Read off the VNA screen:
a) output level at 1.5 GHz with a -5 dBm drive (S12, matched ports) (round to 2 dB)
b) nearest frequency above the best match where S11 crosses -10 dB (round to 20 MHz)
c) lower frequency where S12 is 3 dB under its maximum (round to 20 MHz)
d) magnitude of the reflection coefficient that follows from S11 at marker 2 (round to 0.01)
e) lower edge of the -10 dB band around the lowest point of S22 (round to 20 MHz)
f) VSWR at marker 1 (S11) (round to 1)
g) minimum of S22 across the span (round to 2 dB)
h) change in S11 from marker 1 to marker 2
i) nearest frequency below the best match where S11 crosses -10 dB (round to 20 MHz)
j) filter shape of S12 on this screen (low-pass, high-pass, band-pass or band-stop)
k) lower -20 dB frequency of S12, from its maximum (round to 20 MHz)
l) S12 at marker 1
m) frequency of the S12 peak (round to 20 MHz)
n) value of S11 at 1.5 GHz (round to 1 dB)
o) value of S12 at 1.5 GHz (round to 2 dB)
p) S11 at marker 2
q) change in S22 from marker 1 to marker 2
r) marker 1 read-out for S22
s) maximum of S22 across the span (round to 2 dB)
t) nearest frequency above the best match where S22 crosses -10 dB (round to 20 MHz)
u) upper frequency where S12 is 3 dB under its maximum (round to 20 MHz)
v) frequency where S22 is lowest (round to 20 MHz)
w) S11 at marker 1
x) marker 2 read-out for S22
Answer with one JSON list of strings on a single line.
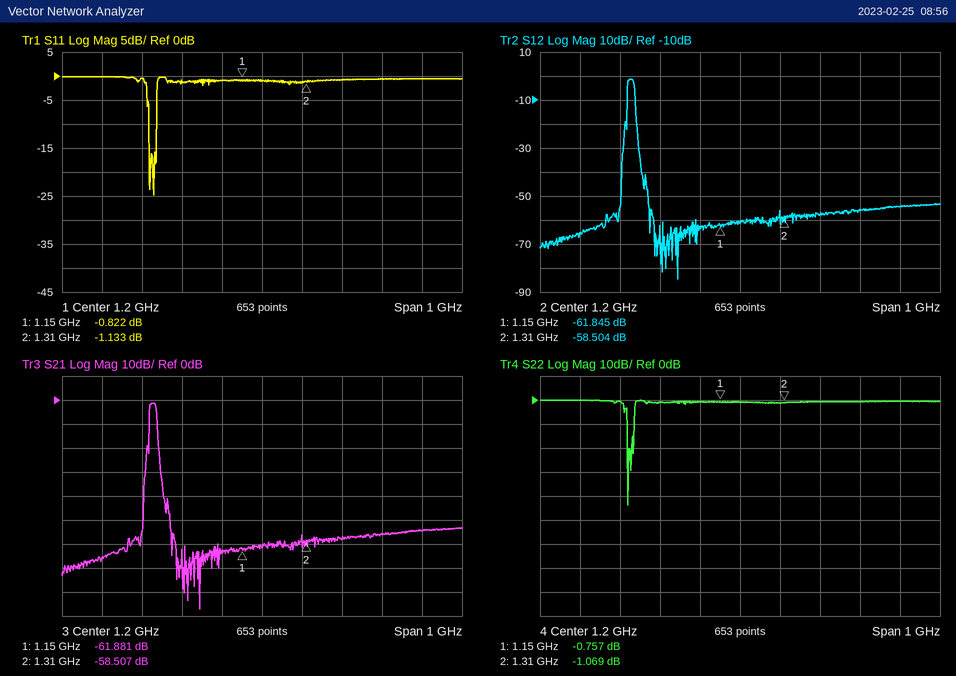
["-60 dBm", "940 MHz", "920 MHz", "0.88", "920 MHz", "21", "-44 dB", "-0.311 dB", "920 MHz", "band-pass", "920 MHz", "-61.845 dB", "920 MHz", "-1 dB", "-56 dB", "-1.133 dB", "-0.312 dB", "-0.757 dB", "0 dB", "940 MHz", "940 MHz", "920 MHz", "-0.822 dB", "-1.069 dB"]
